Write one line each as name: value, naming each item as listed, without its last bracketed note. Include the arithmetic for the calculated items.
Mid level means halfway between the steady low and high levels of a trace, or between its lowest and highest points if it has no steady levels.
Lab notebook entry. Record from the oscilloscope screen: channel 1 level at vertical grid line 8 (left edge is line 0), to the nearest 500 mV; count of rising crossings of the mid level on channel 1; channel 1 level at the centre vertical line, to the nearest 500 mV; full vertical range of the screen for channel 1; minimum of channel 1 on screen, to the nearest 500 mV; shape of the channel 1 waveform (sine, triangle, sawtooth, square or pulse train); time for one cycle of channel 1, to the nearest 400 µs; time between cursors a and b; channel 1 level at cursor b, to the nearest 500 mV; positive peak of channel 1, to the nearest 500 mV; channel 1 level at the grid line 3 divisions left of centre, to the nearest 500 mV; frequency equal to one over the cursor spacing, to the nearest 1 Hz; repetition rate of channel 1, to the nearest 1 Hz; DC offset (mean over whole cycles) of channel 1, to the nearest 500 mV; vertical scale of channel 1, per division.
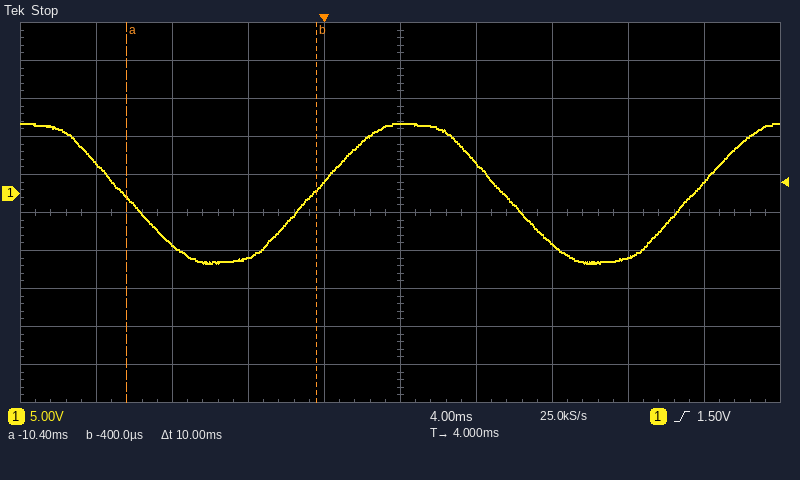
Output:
channel 1 level at vertical grid line 8 (left edge is line 0), to the nearest 500 mV: -8.5 V
count of rising crossings of the mid level on channel 1: 2
channel 1 level at the centre vertical line, to the nearest 500 mV: 9.0 V
full vertical range of the screen for channel 1: 50 V
minimum of channel 1 on screen, to the nearest 500 mV: -9.0 V
shape of the channel 1 waveform: sine
time for one cycle of channel 1, to the nearest 400 µs: 20.0 ms
time between cursors a and b: 10 ms
channel 1 level at cursor b, to the nearest 500 mV: 500 mV
positive peak of channel 1, to the nearest 500 mV: 9.0 V
channel 1 level at the grid line 3 divisions left of centre, to the nearest 500 mV: -6.5 V
frequency equal to one over the cursor spacing, to the nearest 1 Hz: 1 / 10 ms ≈ 100 Hz
repetition rate of channel 1, to the nearest 1 Hz: 1 / 20.0 ms ≈ 50 Hz
DC offset (mean over whole cycles) of channel 1, to the nearest 500 mV: (9.0 V + (-9.0 V)) / 2 ≈ 0.0 V
vertical scale of channel 1, per division: 5 V
